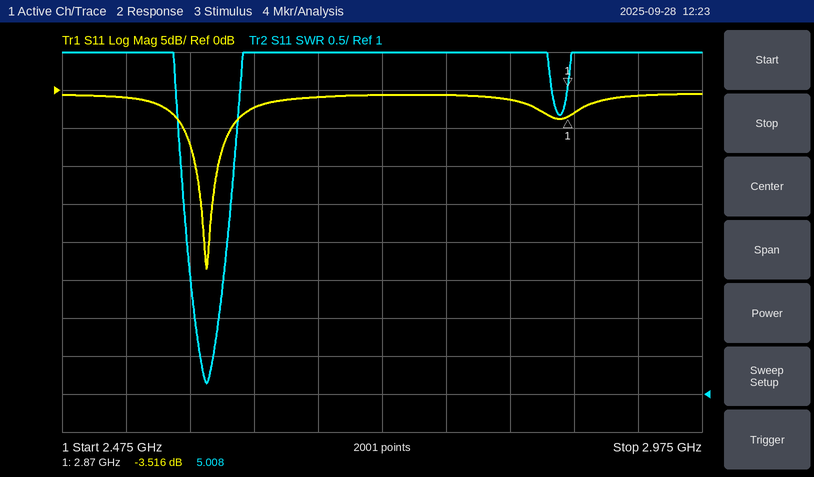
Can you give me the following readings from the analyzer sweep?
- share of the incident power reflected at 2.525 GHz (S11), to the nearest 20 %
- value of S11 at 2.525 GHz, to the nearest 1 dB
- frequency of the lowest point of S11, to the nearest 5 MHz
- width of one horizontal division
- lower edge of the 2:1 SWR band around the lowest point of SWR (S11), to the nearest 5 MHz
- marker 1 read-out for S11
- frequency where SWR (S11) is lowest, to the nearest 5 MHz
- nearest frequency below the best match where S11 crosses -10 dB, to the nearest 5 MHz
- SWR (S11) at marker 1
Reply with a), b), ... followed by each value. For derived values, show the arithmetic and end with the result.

a) 10^(-1/10) ≈ 79.4 %, so 80 % to the nearest 20 %
b) -1 dB
c) 2.590 GHz
d) 50 MHz
e) 2.580 GHz
f) -3.516 dB
g) 2.590 GHz
h) 2.580 GHz
i) 5.008
